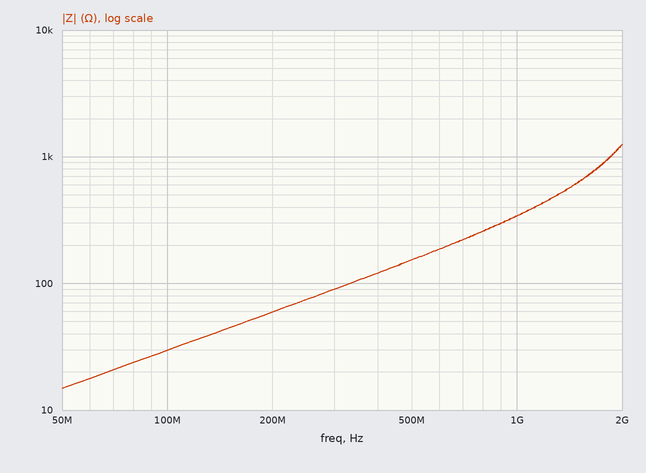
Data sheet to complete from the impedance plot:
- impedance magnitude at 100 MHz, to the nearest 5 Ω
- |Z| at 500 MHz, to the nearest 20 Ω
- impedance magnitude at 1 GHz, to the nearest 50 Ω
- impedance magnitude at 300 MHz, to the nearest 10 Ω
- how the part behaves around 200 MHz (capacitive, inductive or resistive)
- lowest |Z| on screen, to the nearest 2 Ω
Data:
30 Ω
160 Ω
350 Ω
90 Ω
inductive
14 Ω
